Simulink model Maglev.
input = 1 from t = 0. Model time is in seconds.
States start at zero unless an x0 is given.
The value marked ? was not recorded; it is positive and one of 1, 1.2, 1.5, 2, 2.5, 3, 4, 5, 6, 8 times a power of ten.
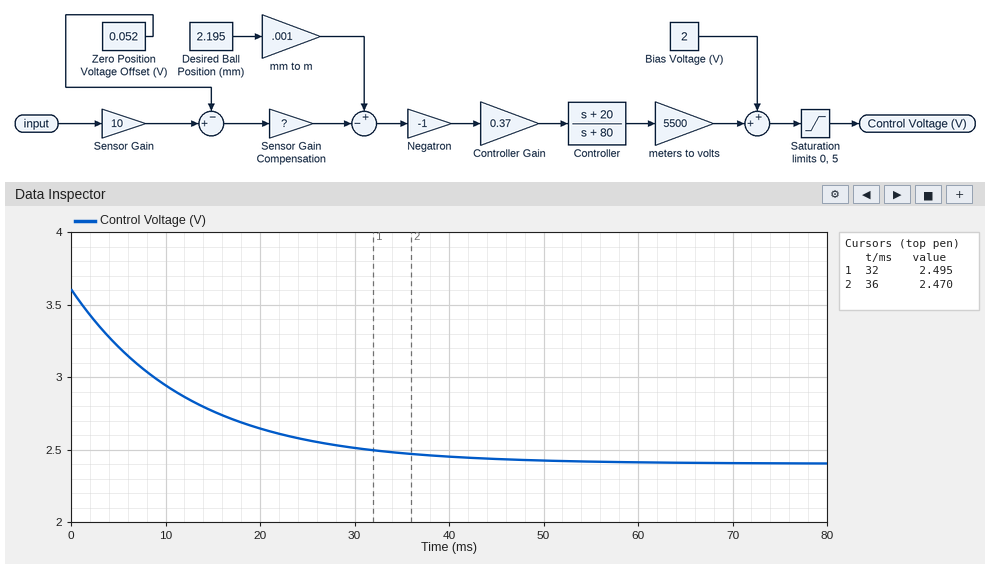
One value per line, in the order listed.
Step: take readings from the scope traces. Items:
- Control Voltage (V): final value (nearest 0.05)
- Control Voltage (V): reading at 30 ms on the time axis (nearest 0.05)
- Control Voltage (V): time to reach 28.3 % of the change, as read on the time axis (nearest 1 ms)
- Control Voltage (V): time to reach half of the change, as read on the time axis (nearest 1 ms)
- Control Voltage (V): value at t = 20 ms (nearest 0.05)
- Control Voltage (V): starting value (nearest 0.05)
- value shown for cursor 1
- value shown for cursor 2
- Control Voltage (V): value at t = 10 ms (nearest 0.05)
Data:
2.40
2.50
4 ms
9 ms
2.65
3.60
2.495
2.470
2.95
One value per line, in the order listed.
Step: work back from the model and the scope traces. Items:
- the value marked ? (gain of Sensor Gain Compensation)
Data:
0.0003
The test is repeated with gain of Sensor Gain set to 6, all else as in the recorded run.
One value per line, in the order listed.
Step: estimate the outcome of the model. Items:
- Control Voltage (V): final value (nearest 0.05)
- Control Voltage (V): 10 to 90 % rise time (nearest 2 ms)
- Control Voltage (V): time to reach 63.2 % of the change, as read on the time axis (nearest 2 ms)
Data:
1.80
28 ms
12 ms
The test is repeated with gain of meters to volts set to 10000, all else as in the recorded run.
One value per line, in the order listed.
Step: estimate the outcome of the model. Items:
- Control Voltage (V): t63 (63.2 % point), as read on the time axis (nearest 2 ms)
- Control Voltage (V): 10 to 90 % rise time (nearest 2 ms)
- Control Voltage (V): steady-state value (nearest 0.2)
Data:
12 ms
28 ms
2.8
